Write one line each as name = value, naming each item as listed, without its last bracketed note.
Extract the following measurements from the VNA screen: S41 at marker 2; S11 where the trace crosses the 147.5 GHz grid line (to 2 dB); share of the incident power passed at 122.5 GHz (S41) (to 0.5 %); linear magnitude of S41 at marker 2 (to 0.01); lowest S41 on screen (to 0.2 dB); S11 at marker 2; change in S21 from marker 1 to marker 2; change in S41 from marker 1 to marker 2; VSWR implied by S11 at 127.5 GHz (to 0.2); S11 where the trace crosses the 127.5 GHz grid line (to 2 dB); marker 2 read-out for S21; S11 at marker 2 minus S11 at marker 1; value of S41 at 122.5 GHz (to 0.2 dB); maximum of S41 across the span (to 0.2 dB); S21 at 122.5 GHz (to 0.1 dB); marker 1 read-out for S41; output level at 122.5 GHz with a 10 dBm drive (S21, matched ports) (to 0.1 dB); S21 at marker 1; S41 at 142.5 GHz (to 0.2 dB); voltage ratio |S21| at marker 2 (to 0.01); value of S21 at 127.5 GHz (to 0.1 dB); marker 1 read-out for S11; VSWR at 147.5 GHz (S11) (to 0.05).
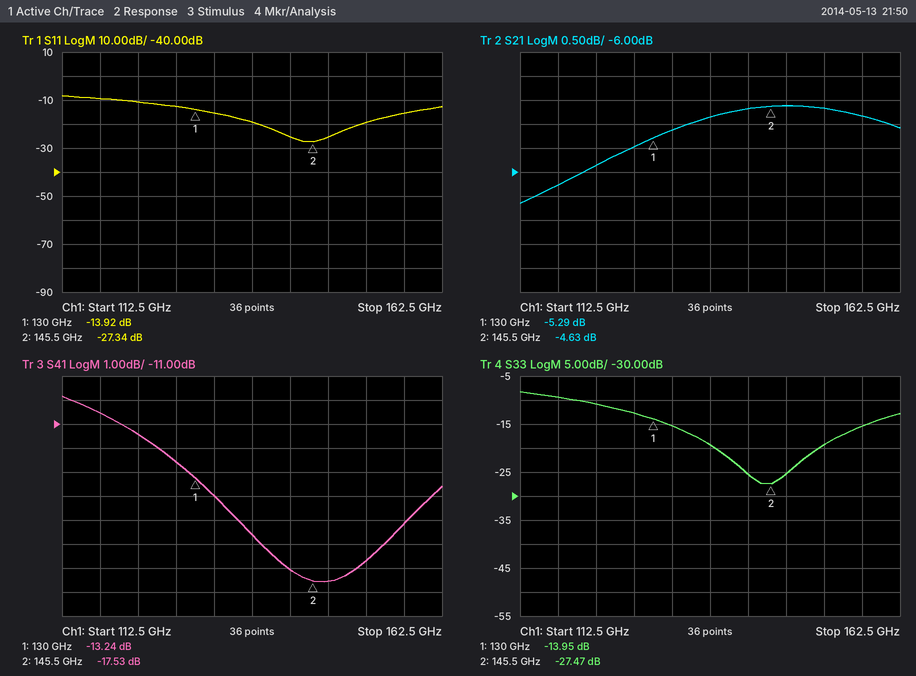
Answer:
S41 at marker 2 = -17.53 dB
S11 where the trace crosses the 147.5 GHz grid line = -26 dB
share of the incident power passed at 122.5 GHz (S41) = 7.0 %
linear magnitude of S41 at marker 2 = 0.13
lowest S41 on screen = -17.6 dB
S11 at marker 2 = -27.34 dB
change in S21 from marker 1 to marker 2 = 0.66 dB
change in S41 from marker 1 to marker 2 = -4.29 dB
VSWR implied by S11 at 127.5 GHz = 1.6
S11 where the trace crosses the 127.5 GHz grid line = -12 dB
marker 2 read-out for S21 = -4.63 dB
S11 at marker 2 minus S11 at marker 1 = -13.42 dB
value of S41 at 122.5 GHz = -11.4 dB
maximum of S41 across the span = -9.8 dB
S21 at 122.5 GHz = -5.9 dB
marker 1 read-out for S41 = -13.24 dB
output level at 122.5 GHz with a 10 dBm drive (S21, matched ports) = 4.1 dBm
S21 at marker 1 = -5.29 dB
S41 at 142.5 GHz = -17.0 dB
voltage ratio |S21| at marker 2 = 0.59
value of S21 at 127.5 GHz = -5.5 dB
marker 1 read-out for S11 = -13.92 dB
VSWR at 147.5 GHz (S11) = 1.10
